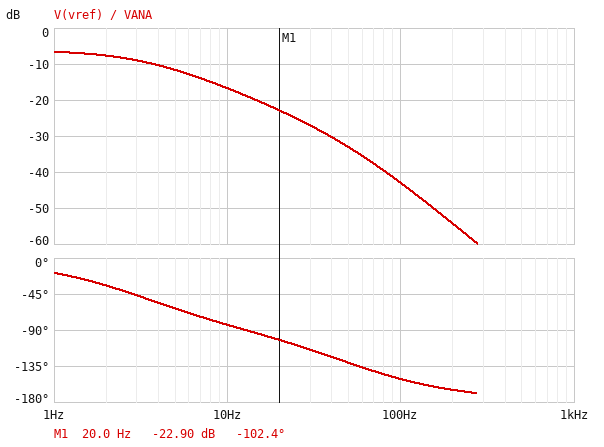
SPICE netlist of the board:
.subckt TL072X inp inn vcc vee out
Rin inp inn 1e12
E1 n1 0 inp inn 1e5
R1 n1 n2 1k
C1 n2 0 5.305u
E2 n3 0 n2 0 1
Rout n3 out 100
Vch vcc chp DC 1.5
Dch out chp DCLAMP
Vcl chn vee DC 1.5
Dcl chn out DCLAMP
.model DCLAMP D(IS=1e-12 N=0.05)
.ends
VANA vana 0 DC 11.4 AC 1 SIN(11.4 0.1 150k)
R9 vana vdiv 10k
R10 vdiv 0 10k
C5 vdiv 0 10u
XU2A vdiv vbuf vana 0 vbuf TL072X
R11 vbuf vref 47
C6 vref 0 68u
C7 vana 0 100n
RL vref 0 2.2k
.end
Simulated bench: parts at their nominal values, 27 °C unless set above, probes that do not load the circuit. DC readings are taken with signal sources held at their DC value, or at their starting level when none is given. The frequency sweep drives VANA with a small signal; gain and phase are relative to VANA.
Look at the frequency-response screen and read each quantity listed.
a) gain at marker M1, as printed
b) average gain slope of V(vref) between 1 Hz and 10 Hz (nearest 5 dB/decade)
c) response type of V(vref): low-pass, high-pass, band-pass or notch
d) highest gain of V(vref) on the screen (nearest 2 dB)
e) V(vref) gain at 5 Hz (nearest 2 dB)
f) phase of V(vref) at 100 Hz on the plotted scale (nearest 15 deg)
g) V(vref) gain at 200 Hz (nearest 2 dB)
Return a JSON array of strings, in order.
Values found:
["-22.90 dB", "-10 dB/decade", "low-pass", "-6 dB", "-12 dB", "-150 deg", "-54 dB"]
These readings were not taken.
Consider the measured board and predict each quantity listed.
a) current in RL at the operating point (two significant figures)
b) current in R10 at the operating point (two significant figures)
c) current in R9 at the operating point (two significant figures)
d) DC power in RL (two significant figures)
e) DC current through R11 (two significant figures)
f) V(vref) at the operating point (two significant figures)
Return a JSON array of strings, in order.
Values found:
["2.5 mA", "570 µA", "570 µA", "14 mW", "2.5 mA", "5.6 V"]
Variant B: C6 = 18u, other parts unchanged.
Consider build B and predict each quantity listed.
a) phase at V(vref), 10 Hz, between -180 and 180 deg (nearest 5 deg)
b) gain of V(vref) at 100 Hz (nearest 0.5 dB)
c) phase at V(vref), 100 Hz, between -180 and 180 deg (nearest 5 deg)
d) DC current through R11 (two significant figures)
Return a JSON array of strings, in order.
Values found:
["-75 deg", "-37.0 dB", "-115 deg", "2.5 mA"]
